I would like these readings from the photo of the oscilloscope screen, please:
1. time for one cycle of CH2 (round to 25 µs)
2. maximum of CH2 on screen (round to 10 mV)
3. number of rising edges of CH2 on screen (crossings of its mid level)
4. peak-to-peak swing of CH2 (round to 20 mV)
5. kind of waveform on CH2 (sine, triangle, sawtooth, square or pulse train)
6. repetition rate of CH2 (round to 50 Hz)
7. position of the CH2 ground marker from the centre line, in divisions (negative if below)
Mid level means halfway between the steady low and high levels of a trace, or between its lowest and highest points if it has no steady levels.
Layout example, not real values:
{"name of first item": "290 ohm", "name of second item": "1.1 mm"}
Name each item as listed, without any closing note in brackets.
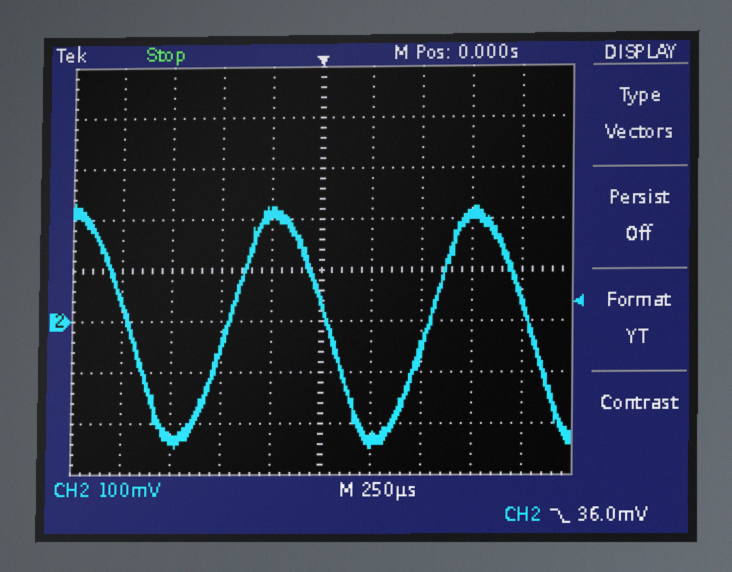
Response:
{"time for one cycle of CH2": "1.000 ms", "maximum of CH2 on screen": "230 mV", "number of rising edges of CH2 on screen": "2", "peak-to-peak swing of CH2": "480 mV", "kind of waveform on CH2": "sine", "repetition rate of CH2": "1.00 kHz", "position of the CH2 ground marker from the centre line, in divisions": "-1.0 div"}
